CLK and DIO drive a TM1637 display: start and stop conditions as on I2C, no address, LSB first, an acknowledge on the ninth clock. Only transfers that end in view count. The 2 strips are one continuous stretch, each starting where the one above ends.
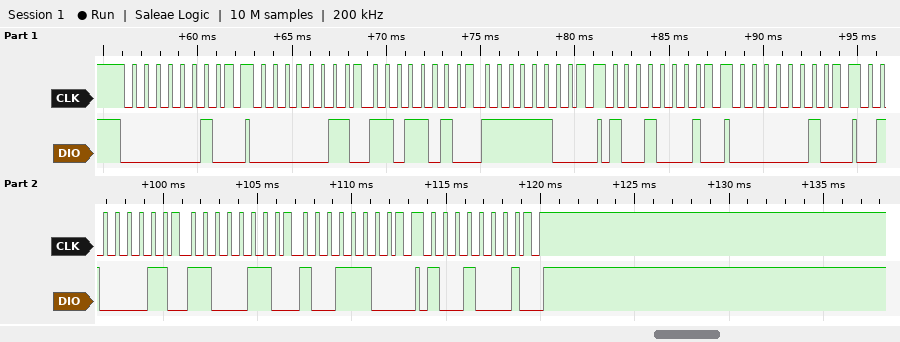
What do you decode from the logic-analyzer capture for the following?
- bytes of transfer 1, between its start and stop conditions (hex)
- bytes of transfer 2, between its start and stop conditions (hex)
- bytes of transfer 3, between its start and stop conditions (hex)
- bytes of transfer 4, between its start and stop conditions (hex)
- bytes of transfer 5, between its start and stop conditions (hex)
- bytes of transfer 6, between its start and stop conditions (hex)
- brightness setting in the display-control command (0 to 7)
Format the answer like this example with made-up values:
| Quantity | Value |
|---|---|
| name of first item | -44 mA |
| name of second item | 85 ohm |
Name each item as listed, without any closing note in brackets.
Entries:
| Quantity | Value |
|---|---|
| bytes of transfer 1, between its start and stop conditions | 40 |
| bytes of transfer 2, between its start and stop conditions | C0 5B 3F |
| bytes of transfer 3, between its start and stop conditions | 89 |
| bytes of transfer 4, between its start and stop conditions | 40 |
| bytes of transfer 5, between its start and stop conditions | C2 63 39 |
| bytes of transfer 6, between its start and stop conditions | 89 |
| brightness setting in the display-control command | 1 |
